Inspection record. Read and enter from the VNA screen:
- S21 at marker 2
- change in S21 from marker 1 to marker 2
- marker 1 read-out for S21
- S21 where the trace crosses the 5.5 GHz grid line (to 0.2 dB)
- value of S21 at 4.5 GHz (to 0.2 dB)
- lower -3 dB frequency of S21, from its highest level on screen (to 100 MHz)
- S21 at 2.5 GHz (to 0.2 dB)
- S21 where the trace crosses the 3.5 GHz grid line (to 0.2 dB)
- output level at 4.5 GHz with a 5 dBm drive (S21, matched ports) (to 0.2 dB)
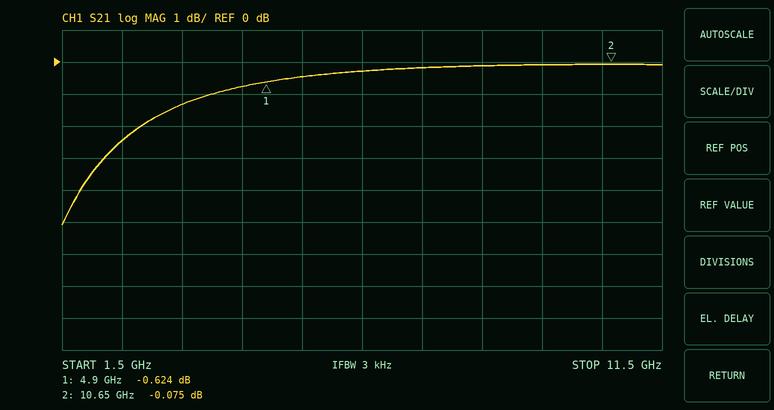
-0.075 dB
0.549 dB
-0.624 dB
-0.4 dB
-0.8 dB
2.2 GHz
-2.4 dB
-1.4 dB
4.2 dBm
